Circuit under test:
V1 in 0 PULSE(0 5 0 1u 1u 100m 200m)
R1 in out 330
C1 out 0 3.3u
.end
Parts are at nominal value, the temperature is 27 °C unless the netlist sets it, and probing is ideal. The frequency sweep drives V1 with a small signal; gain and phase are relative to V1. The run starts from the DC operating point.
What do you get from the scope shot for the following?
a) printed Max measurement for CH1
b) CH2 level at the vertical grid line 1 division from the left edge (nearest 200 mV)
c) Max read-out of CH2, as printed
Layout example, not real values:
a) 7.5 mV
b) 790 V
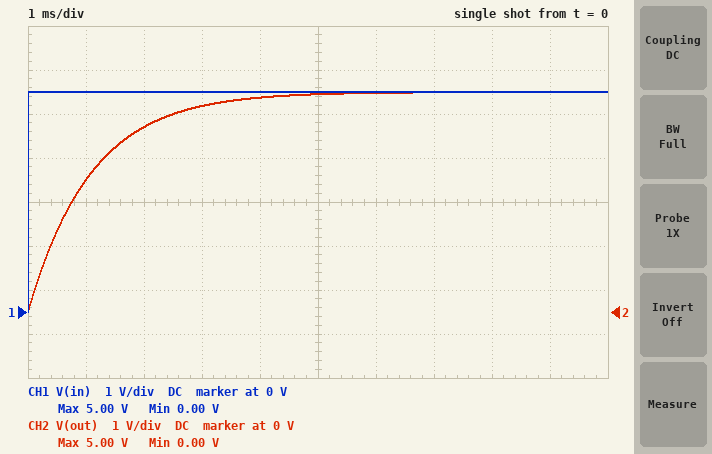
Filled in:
a) 5.00 V
b) 3.0 V
c) 5.00 V
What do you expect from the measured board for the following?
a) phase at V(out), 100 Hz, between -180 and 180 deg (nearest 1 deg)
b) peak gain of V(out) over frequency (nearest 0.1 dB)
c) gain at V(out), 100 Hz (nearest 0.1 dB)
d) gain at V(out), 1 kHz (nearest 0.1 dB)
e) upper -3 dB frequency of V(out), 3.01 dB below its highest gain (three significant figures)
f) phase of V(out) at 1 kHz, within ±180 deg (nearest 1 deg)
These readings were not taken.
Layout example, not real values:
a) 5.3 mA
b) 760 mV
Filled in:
a) -34 deg
b) 0 dB
c) -1.7 dB
d) -16.8 dB
e) 146 Hz
f) -82 deg
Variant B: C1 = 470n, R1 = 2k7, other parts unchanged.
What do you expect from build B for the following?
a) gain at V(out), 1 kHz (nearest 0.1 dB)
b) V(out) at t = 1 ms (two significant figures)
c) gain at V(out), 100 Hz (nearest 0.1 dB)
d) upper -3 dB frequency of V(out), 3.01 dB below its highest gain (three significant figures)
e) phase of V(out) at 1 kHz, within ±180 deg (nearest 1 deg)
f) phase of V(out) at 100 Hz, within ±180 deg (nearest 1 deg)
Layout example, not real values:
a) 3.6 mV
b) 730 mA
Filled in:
a) -18.1 dB
b) 2.7 V
c) -2.1 dB
d) 125 Hz
e) -83 deg
f) -39 deg
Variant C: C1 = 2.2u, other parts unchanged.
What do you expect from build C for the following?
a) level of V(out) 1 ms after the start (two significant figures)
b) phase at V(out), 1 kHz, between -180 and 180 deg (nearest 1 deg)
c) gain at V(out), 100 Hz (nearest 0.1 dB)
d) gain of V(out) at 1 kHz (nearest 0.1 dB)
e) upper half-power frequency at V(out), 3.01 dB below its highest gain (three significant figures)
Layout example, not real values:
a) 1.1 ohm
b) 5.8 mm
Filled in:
a) 3.7 V
b) -78 deg
c) -0.8 dB
d) -13.4 dB
e) 219 Hz
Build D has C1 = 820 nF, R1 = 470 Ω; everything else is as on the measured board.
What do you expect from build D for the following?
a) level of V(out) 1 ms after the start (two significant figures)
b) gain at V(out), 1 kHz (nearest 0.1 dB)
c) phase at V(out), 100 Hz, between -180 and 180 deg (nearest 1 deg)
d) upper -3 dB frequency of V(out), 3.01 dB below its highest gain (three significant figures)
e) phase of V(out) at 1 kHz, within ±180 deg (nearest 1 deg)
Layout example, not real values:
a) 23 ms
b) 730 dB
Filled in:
a) 4.6 V
b) -8.4 dB
c) -14 deg
d) 413 Hz
e) -68 deg
